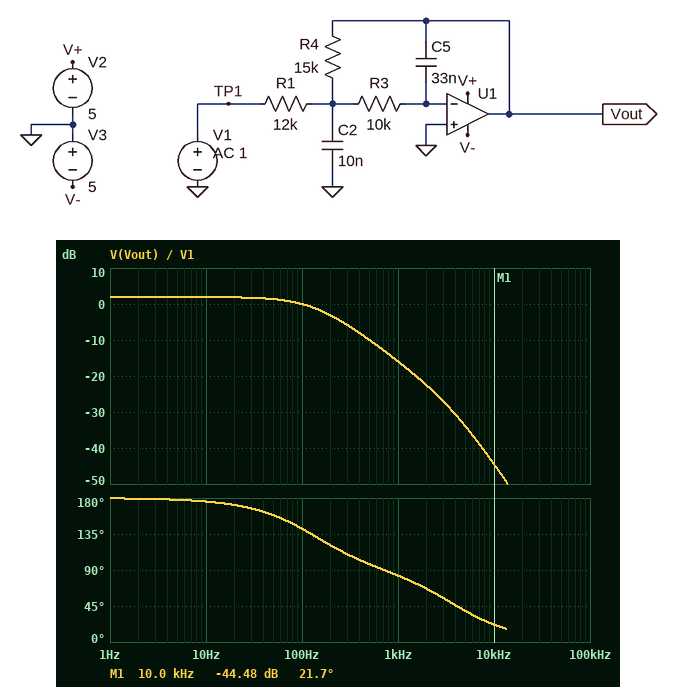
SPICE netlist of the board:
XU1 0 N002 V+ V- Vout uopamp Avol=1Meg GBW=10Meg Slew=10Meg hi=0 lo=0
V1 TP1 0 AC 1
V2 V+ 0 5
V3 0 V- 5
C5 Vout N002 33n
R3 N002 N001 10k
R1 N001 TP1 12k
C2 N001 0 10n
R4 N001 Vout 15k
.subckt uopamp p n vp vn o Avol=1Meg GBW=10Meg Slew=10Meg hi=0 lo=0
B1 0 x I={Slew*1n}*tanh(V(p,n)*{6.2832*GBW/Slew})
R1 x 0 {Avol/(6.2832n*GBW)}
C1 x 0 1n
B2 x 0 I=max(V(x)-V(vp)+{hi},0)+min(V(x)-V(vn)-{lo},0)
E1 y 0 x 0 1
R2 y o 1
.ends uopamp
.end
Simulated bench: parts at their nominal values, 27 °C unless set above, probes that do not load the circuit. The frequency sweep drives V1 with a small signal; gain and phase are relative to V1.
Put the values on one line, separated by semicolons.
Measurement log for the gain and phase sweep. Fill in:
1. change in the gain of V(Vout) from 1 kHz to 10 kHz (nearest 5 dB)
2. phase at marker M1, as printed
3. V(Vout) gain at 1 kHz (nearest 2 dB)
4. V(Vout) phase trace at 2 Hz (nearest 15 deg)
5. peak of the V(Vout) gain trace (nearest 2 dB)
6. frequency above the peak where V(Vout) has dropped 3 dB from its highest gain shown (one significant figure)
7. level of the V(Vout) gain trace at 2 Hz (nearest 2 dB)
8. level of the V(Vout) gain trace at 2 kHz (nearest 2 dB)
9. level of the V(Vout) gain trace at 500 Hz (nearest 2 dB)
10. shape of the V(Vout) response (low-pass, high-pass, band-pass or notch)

-30 dB; 21.7 deg; -16 dB; 180 deg; 2 dB; 100 Hz; 2 dB; -22 dB; -10 dB; low-pass
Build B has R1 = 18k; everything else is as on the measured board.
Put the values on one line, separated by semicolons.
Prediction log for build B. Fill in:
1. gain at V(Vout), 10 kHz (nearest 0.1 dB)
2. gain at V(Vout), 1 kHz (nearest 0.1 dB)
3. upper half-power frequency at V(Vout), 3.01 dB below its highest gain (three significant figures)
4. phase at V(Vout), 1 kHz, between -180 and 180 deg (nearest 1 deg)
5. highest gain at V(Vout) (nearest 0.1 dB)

-47.9 dB; -18.5 dB; 151 Hz; 82 deg; -1.6 dB
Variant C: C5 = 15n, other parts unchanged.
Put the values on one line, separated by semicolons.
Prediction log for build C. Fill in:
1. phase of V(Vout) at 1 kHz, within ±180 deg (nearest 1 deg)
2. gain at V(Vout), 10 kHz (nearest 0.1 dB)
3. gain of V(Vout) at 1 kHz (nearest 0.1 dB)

92 deg; -37.6 dB; -9.0 dB
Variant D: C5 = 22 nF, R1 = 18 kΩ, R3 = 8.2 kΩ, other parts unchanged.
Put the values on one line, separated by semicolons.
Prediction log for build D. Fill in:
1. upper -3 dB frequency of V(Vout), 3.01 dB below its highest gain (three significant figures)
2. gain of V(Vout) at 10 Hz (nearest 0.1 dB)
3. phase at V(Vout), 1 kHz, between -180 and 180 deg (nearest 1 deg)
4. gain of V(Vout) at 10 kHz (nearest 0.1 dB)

257 Hz; -1.6 dB; 89 deg; -42.7 dB
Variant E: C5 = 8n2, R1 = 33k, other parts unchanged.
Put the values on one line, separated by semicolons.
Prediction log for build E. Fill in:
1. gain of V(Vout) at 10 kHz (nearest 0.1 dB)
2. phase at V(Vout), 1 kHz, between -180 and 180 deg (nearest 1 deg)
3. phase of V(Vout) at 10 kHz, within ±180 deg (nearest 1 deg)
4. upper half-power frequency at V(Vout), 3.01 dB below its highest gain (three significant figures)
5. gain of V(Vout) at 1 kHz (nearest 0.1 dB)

-40.8 dB; 109 deg; 18 deg; 816 Hz; -11.0 dB
